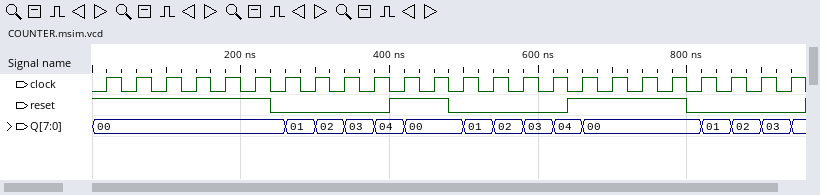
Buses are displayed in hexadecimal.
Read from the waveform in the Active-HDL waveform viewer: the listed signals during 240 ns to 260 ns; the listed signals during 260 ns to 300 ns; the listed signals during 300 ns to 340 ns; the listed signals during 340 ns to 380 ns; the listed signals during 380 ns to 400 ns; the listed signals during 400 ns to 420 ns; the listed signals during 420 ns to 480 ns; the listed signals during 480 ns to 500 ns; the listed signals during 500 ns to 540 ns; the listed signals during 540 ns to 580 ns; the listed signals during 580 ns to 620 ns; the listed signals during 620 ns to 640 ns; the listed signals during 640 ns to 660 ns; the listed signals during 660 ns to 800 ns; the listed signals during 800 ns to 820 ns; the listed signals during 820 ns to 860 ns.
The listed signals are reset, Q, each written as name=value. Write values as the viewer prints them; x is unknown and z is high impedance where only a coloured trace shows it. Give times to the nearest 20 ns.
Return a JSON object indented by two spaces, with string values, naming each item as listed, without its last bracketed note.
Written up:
{
  "the listed signals during 240 ns to 260 ns": "reset=0, Q=00",
  "the listed signals during 260 ns to 300 ns": "reset=0, Q=01",
  "the listed signals during 300 ns to 340 ns": "reset=0, Q=02",
  "the listed signals during 340 ns to 380 ns": "reset=0, Q=03",
  "the listed signals during 380 ns to 400 ns": "reset=0, Q=04",
  "the listed signals during 400 ns to 420 ns": "reset=1, Q=04",
  "the listed signals during 420 ns to 480 ns": "reset=1, Q=00",
  "the listed signals during 480 ns to 500 ns": "reset=0, Q=00",
  "the listed signals during 500 ns to 540 ns": "reset=0, Q=01",
  "the listed signals during 540 ns to 580 ns": "reset=0, Q=02",
  "the listed signals during 580 ns to 620 ns": "reset=0, Q=03",
  "the listed signals during 620 ns to 640 ns": "reset=0, Q=04",
  "the listed signals during 640 ns to 660 ns": "reset=1, Q=04",
  "the listed signals during 660 ns to 800 ns": "reset=1, Q=00",
  "the listed signals during 800 ns to 820 ns": "reset=0, Q=00",
  "the listed signals during 820 ns to 860 ns": "reset=0, Q=01"
}
